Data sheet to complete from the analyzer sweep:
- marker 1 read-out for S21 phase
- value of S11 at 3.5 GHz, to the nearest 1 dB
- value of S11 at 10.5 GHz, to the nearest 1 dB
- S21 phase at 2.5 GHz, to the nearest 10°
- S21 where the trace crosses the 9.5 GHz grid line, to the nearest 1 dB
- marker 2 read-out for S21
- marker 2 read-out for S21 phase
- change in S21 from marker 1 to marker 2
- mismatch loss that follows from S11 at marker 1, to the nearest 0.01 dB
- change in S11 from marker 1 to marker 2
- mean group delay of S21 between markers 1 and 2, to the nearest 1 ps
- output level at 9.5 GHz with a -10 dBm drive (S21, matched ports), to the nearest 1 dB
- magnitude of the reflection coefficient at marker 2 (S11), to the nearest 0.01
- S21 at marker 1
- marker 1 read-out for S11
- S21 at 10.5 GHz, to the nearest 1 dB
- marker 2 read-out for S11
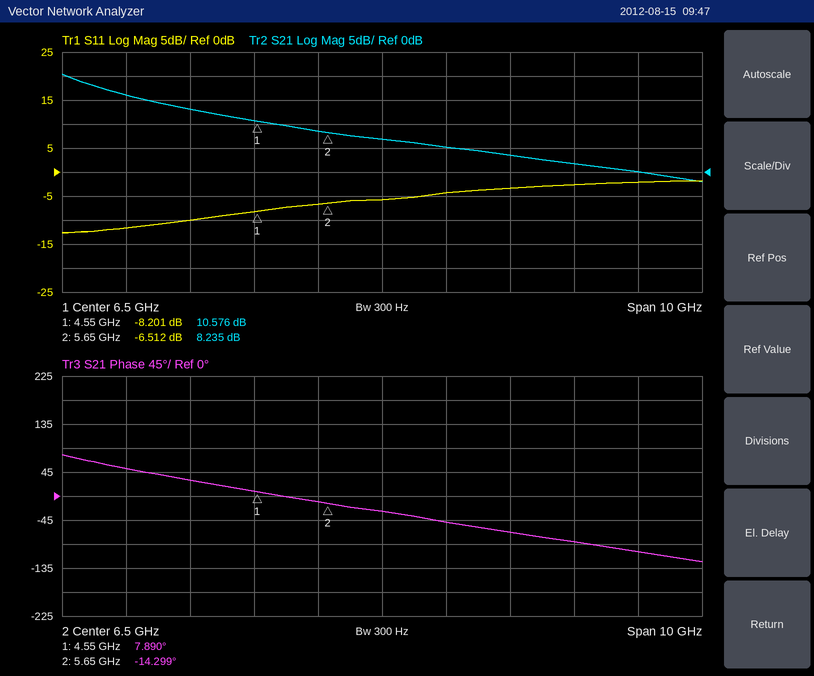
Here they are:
7.890°
-10 dB
-2 dB
50°
2 dB
8.235 dB
-14.299°
-2.341 dB
0.71 dB
1.689 dB
56 ps
-8 dBm
0.47
10.576 dB
-8.201 dB
0 dB
-6.512 dB
